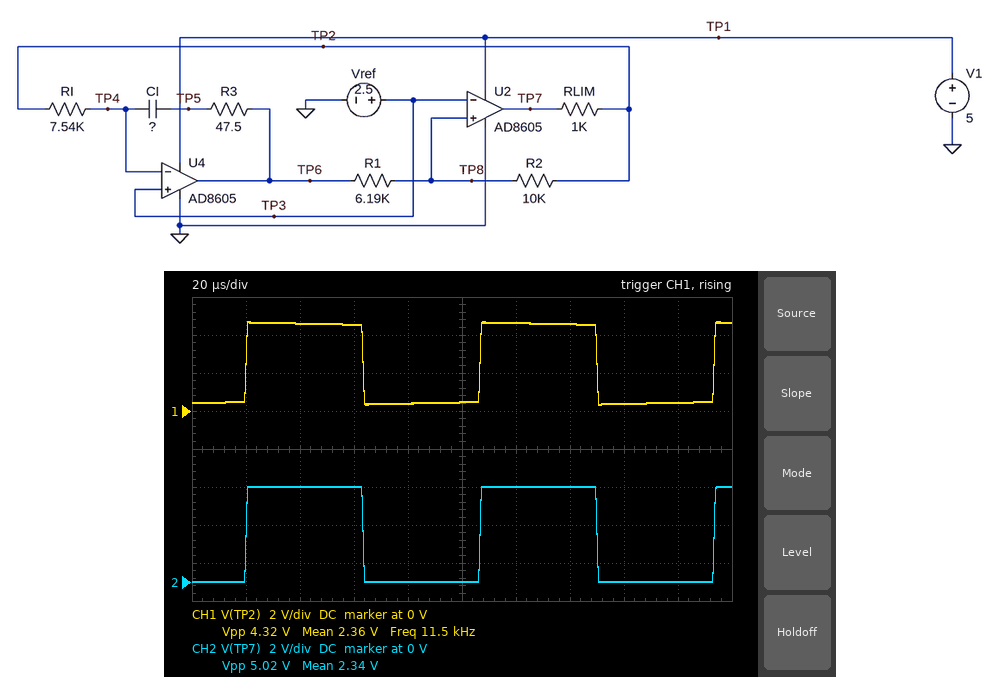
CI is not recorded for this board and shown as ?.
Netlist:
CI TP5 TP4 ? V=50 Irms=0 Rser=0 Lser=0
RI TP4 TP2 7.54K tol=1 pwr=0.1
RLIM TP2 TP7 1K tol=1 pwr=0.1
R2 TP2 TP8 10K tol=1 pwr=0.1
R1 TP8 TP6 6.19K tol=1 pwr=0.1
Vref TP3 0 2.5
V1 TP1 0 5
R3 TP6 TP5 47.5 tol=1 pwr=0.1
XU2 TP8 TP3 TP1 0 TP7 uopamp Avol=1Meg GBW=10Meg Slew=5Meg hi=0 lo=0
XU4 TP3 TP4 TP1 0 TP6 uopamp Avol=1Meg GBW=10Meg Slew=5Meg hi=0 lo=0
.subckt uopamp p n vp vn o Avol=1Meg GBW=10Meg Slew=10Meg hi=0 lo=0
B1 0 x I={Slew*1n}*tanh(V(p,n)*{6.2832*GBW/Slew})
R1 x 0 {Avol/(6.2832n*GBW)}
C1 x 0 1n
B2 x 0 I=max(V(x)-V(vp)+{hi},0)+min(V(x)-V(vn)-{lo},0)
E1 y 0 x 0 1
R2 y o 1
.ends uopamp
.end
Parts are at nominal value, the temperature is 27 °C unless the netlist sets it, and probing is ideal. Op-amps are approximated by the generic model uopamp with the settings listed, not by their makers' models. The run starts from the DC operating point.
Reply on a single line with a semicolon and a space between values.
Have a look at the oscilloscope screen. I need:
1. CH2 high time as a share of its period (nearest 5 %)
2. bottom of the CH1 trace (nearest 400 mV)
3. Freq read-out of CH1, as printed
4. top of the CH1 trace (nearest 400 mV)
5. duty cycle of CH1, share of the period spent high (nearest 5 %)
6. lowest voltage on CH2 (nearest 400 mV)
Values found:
50 %; 400 mV; 11.5 kHz; 4.8 V; 50 %; 0 V
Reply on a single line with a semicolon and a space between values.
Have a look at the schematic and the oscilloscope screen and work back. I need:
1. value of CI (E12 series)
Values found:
4.7 nF
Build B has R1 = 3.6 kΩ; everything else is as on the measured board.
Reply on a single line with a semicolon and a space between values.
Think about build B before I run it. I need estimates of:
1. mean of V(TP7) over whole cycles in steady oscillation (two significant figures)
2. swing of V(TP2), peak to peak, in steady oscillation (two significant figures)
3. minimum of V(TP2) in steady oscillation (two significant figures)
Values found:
2.5 V; 4.2 V; 380 mV
